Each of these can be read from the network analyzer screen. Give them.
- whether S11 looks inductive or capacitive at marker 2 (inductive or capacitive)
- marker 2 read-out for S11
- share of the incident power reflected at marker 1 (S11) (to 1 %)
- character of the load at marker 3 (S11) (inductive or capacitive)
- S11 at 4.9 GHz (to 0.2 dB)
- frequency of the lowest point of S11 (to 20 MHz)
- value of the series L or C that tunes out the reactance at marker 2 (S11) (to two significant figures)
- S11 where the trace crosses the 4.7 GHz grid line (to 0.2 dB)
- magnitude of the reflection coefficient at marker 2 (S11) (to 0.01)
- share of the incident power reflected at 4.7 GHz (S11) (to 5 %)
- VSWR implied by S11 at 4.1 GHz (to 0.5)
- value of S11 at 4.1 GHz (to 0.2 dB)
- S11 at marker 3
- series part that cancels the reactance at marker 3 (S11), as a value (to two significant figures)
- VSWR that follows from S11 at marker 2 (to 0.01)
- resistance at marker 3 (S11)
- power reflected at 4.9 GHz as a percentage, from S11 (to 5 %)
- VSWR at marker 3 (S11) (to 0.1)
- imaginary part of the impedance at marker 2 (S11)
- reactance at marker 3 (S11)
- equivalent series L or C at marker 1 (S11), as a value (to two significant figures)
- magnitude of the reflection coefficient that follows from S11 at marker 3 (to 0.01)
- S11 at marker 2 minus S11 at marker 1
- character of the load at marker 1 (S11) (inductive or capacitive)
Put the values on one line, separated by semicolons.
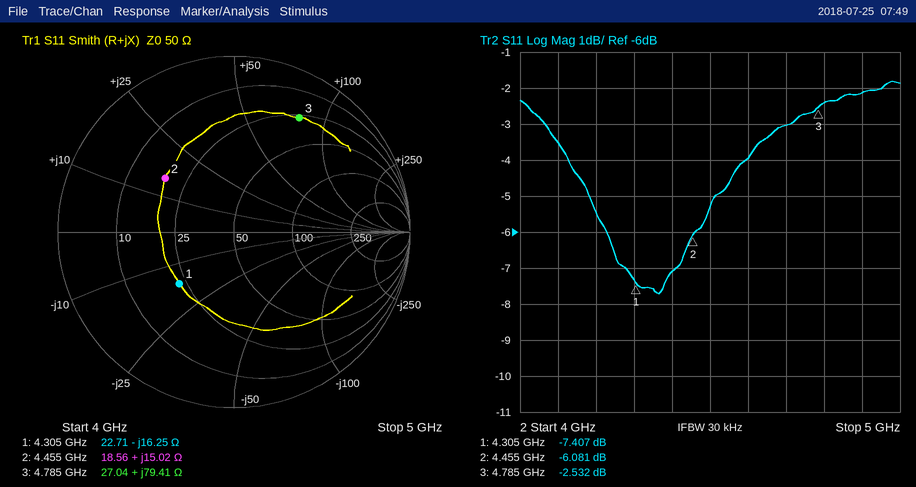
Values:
inductive; -6.081 dB; 18 %; inductive; -2.2 dB; 4.36 GHz; 2.4 pF; -3.0 dB; 0.50; 50 %; 5.0; -3.6 dB; -2.532 dB; 420 fF; 2.97; 27.04 Ω; 60 %; 6.9; +15.02 Ω; +79.41 Ω; 2.3 pF; 0.75; 1.326 dB; capacitive
